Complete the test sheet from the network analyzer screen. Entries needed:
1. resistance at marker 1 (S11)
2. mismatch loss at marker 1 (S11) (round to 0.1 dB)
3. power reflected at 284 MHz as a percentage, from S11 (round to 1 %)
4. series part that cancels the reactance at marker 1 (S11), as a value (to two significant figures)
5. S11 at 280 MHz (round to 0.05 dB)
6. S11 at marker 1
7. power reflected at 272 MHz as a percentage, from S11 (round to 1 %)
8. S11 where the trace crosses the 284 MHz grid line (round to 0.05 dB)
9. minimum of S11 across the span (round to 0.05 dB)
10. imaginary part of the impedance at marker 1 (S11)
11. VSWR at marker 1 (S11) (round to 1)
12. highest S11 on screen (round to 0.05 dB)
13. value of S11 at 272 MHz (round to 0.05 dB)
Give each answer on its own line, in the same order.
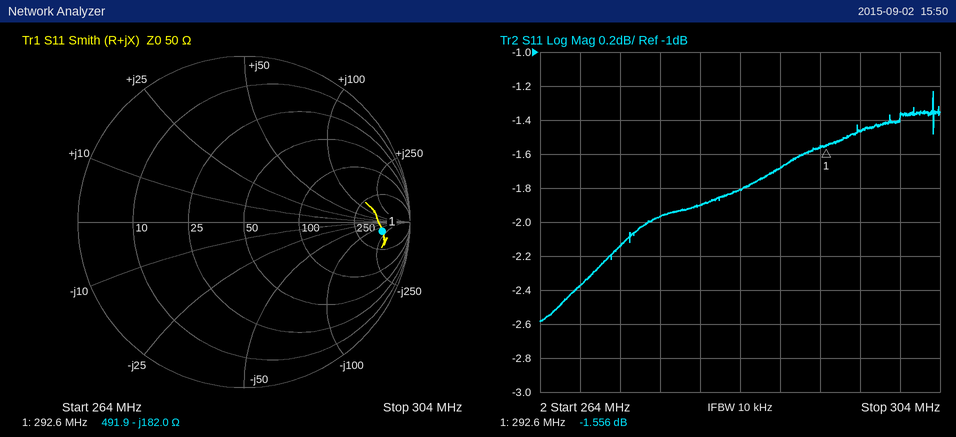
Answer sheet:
491.9 Ω
5.2 dB
66 %
99 nH
-1.90 dB
-1.556 dB
61 %
-1.80 dB
-2.60 dB
-182.0 Ω
11
-1.25 dB
-2.15 dB
